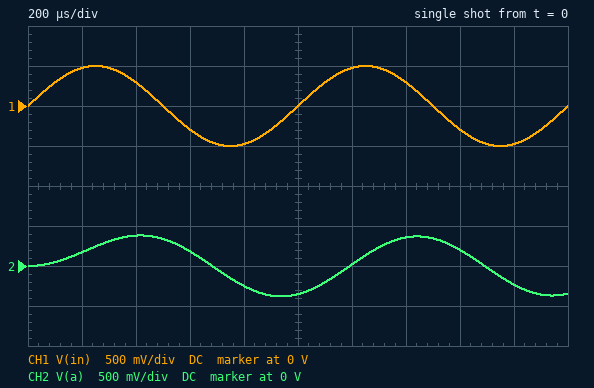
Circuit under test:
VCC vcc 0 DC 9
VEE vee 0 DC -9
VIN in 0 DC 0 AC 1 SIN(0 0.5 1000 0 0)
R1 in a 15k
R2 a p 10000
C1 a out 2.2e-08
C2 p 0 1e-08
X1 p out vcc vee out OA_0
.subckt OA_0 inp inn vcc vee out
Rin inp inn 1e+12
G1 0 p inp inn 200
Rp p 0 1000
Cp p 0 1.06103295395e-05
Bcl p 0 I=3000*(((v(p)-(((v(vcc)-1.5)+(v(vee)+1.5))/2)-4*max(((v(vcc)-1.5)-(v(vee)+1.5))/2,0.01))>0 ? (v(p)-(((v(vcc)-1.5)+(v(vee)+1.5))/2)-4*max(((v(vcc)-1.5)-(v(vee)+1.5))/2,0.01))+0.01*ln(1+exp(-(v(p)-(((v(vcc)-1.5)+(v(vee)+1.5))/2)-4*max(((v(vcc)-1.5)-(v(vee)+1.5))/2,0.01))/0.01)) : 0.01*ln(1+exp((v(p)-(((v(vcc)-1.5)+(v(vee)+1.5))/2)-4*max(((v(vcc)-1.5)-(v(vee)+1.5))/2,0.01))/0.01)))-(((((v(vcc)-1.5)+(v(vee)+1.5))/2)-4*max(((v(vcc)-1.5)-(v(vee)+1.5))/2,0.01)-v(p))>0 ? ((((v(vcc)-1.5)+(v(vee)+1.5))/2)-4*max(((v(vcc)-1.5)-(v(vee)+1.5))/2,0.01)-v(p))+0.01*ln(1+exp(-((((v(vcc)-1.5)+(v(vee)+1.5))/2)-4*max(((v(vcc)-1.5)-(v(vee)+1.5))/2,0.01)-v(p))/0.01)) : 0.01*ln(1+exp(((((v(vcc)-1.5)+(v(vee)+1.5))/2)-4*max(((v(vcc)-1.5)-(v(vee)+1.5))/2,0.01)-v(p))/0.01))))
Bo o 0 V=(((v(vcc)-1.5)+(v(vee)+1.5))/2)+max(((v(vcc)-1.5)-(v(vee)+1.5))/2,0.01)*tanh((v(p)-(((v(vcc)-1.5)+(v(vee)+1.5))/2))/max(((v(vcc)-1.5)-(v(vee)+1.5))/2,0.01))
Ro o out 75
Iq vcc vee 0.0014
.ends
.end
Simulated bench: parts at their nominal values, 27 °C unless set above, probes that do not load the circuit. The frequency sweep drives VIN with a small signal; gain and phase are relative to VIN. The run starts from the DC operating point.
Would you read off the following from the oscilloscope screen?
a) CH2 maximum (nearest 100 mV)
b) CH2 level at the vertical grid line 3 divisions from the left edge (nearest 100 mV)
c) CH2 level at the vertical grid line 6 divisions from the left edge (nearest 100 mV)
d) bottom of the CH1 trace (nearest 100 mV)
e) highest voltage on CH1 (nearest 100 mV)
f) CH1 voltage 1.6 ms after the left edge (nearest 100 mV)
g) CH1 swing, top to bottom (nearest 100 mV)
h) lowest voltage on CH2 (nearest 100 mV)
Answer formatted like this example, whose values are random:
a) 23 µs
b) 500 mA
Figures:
a) 400 mV
b) 200 mV
c) 0 V
d) -500 mV
e) 500 mV
f) -300 mV
g) 1.0 V
h) -400 mV
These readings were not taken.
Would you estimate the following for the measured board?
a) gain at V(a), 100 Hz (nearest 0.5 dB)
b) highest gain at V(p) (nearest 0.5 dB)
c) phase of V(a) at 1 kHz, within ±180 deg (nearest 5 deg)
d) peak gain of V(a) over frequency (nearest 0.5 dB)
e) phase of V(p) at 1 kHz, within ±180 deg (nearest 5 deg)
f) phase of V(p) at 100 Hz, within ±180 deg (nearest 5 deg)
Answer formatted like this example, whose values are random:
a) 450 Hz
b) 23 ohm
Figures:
a) 0 dB
b) 0 dB
c) -70 deg
d) 0 dB
e) -100 deg
f) -10 deg
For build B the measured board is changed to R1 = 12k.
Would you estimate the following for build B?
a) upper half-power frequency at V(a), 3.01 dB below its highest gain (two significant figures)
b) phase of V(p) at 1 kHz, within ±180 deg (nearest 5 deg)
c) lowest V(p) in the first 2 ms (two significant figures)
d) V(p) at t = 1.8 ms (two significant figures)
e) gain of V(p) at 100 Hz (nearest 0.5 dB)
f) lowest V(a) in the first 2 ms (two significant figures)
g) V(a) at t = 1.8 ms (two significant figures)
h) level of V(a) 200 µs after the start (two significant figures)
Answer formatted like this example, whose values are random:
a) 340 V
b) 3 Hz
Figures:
a) 1.2 kHz
b) -90 deg
c) -370 mV
d) -100 mV
e) 0 dB
f) -430 mV
g) -320 mV
h) 200 mV
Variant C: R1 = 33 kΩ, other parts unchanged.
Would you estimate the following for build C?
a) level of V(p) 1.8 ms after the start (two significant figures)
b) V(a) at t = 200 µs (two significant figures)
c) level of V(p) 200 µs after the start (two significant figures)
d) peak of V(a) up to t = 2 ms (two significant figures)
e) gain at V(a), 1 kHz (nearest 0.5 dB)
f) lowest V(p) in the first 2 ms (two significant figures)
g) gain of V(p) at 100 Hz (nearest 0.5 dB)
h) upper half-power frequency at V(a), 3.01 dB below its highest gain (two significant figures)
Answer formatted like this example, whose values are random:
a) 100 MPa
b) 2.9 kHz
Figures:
a) 42 mV
b) 89 mV
c) 39 mV
d) 250 mV
e) -9.0 dB
f) -150 mV
g) 0 dB
h) 550 Hz
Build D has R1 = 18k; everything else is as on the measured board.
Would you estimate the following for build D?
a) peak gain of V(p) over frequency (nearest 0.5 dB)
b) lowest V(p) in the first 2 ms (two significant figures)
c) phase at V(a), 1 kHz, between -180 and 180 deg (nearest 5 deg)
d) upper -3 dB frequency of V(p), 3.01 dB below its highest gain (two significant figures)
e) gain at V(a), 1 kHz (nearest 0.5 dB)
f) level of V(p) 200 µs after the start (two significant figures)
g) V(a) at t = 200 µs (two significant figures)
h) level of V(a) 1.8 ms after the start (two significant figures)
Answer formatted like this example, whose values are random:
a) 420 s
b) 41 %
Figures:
a) 0 dB
b) -280 mV
c) -75 deg
d) 800 Hz
e) -4.0 dB
f) 67 mV
g) 150 mV
h) -170 mV
